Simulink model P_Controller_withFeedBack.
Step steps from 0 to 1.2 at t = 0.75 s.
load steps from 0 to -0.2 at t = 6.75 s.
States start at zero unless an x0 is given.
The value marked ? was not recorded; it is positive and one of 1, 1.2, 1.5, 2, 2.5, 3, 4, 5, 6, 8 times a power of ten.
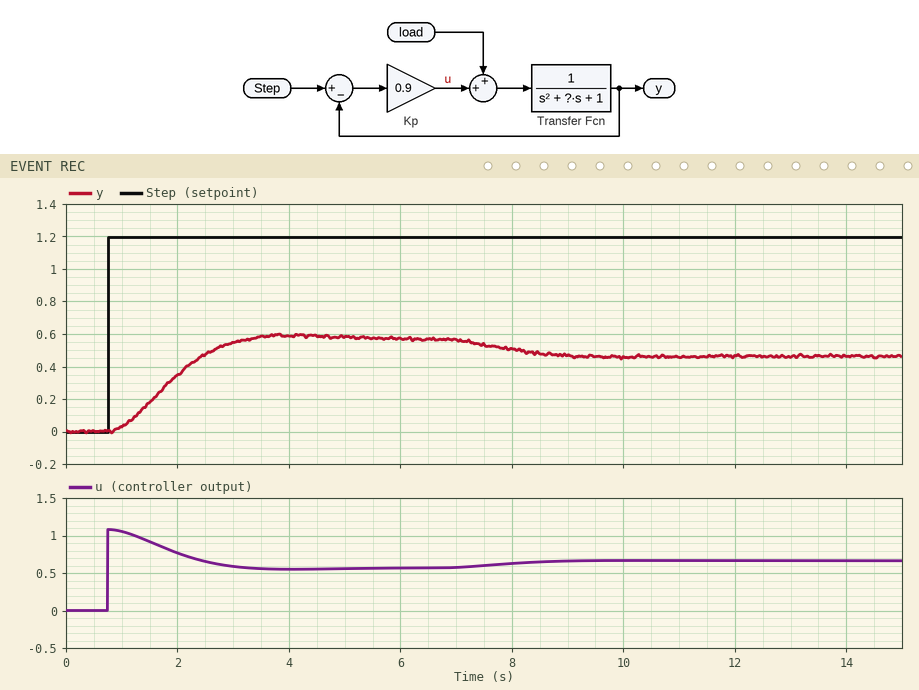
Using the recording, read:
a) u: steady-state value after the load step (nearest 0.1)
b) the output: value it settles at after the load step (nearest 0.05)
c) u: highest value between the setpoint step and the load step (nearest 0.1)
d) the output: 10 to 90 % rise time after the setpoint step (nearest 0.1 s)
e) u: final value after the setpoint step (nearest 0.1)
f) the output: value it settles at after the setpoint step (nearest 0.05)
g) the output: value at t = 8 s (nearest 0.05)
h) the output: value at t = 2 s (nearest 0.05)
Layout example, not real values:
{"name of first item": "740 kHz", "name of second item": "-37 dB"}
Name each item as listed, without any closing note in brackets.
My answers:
{"u: steady-state value after the load step": "0.7", "the output: value it settles at after the load step": "0.45", "u: highest value between the setpoint step and the load step": "1.1", "the output: 10 to 90 % rise time after the setpoint step": "1.6 s", "u: final value after the setpoint step": "0.6", "the output: value it settles at after the setpoint step": "0.55", "the output: value at t = 8 s": "0.50", "the output: value at t = 2 s": "0.35"}
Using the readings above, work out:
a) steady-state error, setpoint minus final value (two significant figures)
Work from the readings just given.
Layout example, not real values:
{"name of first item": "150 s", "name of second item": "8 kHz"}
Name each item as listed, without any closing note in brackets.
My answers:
{"steady-state error, setpoint minus final value": "0.65"}
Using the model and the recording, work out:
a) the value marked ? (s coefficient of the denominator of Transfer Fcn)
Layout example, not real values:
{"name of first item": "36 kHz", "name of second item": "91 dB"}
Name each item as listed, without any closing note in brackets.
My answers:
{"the value marked ?": "2"}
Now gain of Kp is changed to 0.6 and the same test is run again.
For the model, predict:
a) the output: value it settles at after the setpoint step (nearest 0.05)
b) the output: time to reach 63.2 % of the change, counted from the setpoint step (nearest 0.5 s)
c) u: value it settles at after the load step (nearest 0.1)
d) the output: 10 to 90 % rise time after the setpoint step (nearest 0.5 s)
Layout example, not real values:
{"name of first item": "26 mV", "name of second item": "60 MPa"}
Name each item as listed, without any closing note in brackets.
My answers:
{"the output: value it settles at after the setpoint step": "0.45", "the output: time to reach 63.2 % of the change, counted from the setpoint step": "1.5 s", "u: value it settles at after the load step": "0.5", "the output: 10 to 90 % rise time after the setpoint step": "2.0 s"}
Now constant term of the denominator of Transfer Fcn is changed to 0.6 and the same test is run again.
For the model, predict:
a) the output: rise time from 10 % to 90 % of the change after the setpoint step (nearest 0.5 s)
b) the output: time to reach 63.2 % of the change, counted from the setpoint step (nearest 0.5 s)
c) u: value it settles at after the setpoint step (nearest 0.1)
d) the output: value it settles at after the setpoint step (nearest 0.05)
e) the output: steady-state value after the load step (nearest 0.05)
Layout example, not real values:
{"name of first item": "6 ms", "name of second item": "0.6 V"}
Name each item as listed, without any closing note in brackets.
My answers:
{"the output: rise time from 10 % to 90 % of the change after the setpoint step": "2.0 s", "the output: time to reach 63.2 % of the change, counted from the setpoint step": "1.5 s", "u: value it settles at after the setpoint step": "0.4", "the output: value it settles at after the setpoint step": "0.70", "the output: steady-state value after the load step": "0.60"}
